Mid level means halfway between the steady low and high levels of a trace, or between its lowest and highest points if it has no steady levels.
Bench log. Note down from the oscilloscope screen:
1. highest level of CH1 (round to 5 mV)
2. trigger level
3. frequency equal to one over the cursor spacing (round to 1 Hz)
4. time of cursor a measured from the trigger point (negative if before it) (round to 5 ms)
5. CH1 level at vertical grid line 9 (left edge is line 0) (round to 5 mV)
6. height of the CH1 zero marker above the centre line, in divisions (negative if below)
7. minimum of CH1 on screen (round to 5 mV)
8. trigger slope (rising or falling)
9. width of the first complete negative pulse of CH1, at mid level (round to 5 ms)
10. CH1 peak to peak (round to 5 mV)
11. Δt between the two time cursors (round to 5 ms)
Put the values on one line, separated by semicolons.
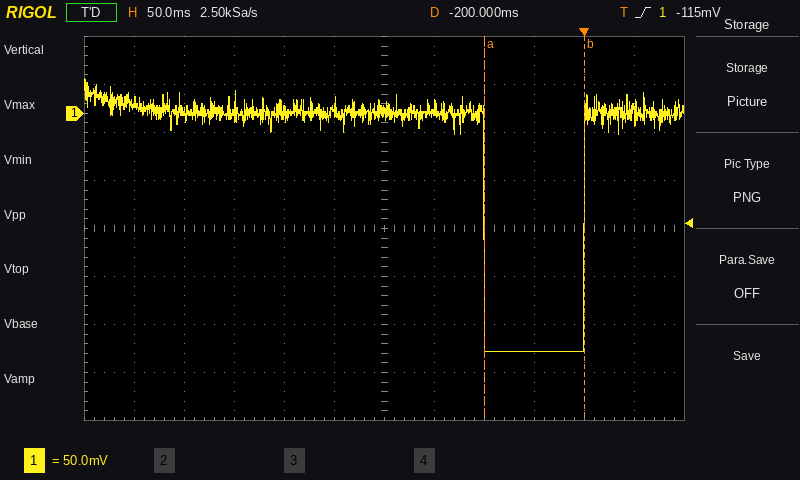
35 mV; -115 mV; 10 Hz; -100 ms; -250 mV; +2.4 div; -250 mV; rising; 100 ms; 285 mV; 100 ms
